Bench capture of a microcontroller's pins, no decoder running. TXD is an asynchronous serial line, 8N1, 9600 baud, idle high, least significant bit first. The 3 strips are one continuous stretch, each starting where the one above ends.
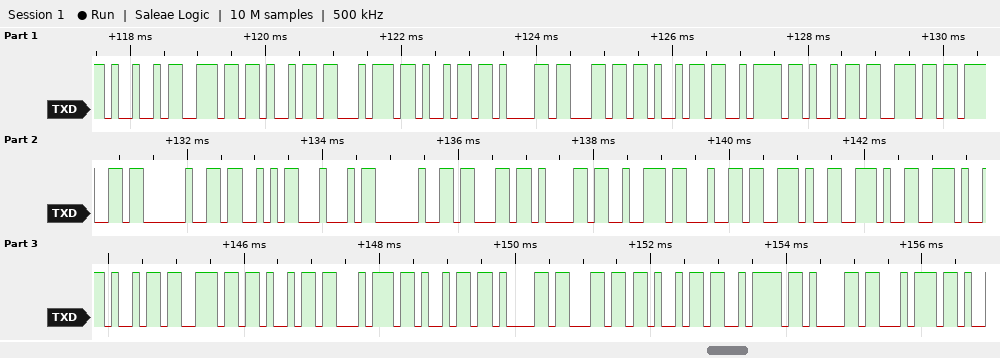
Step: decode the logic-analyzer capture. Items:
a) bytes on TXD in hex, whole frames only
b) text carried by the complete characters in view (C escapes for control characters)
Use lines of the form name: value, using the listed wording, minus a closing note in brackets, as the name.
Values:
bytes on TXD in hex, whole frames only: 49 6E 69 74 69 61 6C 69 7A 69 6E 67 20 53 44 20 63 61 72 64 2E 2E 2E 69 6E 69 74 69 61 6C 69 7A 61 74
text carried by the complete characters in view: "Initializing SD card...initializat"
